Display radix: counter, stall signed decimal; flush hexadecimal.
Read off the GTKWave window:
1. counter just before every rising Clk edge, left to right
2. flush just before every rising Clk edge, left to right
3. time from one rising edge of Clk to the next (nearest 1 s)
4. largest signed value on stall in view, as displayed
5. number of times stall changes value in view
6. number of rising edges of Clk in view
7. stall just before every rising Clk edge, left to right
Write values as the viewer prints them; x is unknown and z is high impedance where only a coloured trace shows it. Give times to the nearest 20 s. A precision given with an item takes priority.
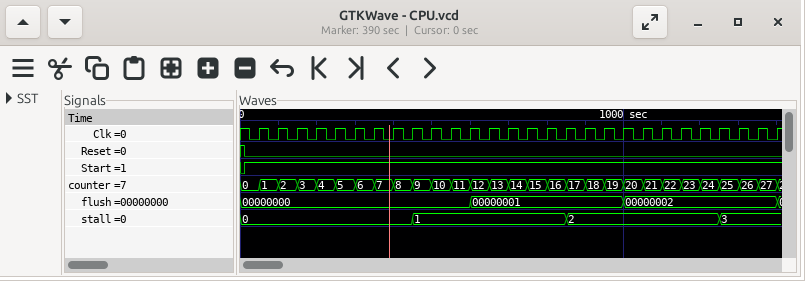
0, 1, 2, 3, 4, 5, 6, 7, 8, 9, 10, 11, 12, 13, 14, 15, 16, 17, 18, 19, 20, 21, 22, 23, 24, 25, 26, 27
00000000, 00000000, 00000000, 00000000, 00000000, 00000000, 00000000, 00000000, 00000000, 00000000, 00000000, 00000000, 00000001, 00000001, 00000001, 00000001, 00000001, 00000001, 00000001, 00000001, 00000002, 00000002, 00000002, 00000002, 00000002, 00000002, 00000002, 00000002
50 s
3
3
28
0, 0, 0, 0, 0, 0, 0, 0, 0, 1, 1, 1, 1, 1, 1, 1, 1, 2, 2, 2, 2, 2, 2, 2, 2, 3, 3, 3
